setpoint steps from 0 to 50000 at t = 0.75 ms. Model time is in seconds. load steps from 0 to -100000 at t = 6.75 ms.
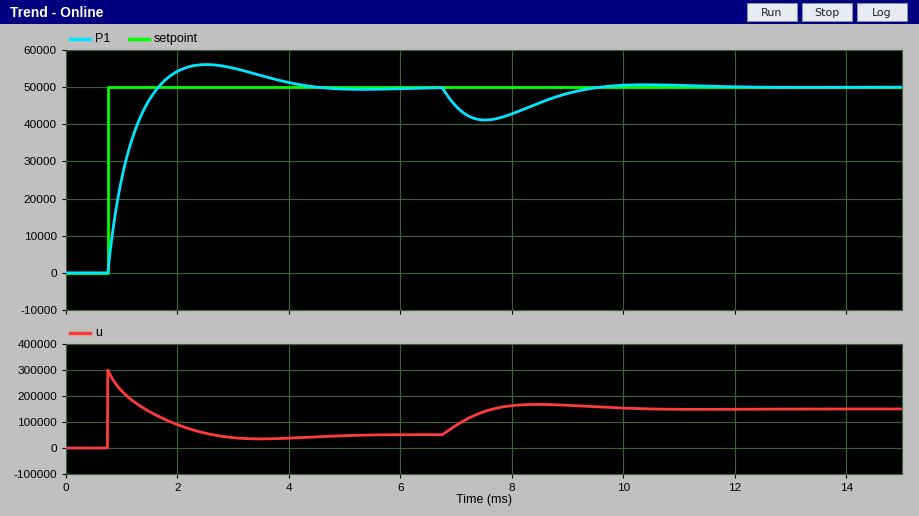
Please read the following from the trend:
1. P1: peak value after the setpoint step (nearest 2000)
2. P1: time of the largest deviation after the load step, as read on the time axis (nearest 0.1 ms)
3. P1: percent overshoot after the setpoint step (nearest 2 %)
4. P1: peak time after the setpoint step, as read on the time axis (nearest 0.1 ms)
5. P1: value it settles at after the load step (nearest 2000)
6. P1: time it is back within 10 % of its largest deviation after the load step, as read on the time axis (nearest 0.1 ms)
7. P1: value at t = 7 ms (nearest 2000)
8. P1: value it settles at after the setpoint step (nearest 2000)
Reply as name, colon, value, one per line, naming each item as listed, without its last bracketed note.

P1: peak value after the setpoint step: 56000
P1: time of the largest deviation after the load step, as read on the time axis: 7.5 ms
P1: percent overshoot after the setpoint step: 12 %
P1: peak time after the setpoint step, as read on the time axis: 2.5 ms
P1: value it settles at after the load step: 50000
P1: time it is back within 10 % of its largest deviation after the load step, as read on the time axis: 9.2 ms
P1: value at t = 7 ms: 44000
P1: value it settles at after the setpoint step: 50000
